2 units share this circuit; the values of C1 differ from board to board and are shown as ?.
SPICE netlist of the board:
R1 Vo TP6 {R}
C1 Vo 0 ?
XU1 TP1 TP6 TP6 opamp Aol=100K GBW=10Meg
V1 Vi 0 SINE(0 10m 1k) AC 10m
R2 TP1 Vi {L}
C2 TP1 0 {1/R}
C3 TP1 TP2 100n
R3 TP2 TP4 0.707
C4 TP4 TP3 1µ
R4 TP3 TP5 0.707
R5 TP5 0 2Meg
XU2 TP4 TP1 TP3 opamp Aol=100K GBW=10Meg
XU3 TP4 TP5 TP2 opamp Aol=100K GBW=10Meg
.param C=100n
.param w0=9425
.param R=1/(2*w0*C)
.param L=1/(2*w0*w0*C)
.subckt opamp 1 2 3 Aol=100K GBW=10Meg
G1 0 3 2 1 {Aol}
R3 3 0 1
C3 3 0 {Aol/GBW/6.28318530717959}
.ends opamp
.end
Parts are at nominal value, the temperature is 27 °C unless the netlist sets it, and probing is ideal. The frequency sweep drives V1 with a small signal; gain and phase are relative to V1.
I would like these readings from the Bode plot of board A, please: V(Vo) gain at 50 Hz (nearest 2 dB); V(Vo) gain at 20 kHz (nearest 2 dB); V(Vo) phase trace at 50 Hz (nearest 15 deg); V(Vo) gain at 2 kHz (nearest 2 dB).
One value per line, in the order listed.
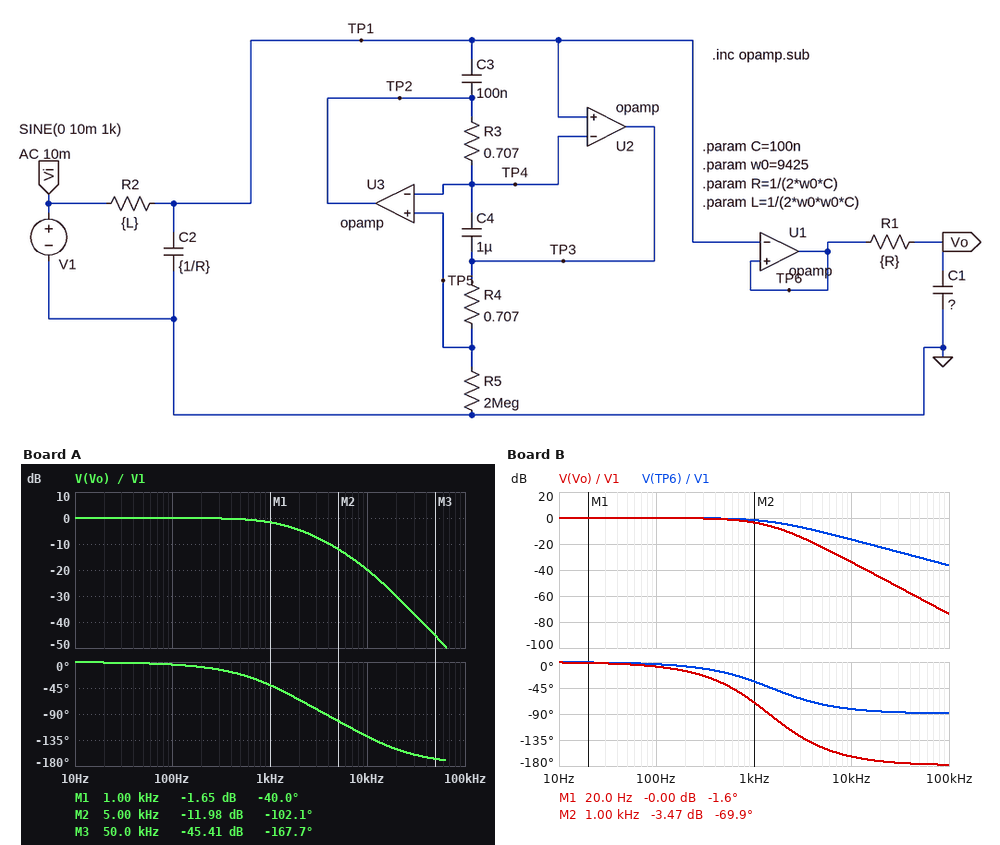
0 dB
-30 dB
0 deg
-4 dB
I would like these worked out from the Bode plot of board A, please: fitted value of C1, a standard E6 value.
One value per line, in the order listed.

33 nF
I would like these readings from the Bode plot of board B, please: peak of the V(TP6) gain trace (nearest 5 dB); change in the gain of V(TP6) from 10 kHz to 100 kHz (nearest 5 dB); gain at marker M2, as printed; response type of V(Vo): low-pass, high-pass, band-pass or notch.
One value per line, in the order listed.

0 dB
-20 dB
-3.47 dB
low-pass
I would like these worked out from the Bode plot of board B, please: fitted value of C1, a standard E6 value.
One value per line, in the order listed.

220 nF
